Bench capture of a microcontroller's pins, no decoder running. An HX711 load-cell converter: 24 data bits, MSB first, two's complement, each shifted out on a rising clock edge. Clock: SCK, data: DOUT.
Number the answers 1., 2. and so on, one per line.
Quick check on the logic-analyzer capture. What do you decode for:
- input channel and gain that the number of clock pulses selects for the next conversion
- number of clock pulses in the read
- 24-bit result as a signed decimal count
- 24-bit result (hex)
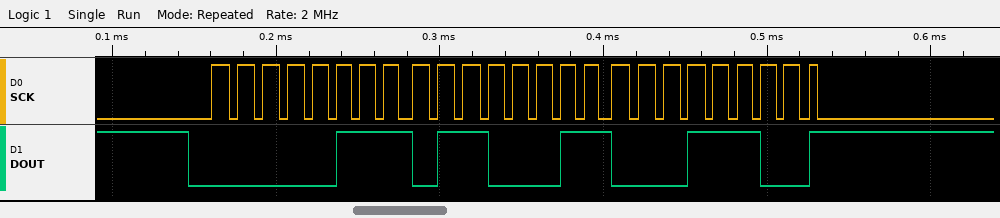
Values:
1. channel A, gain 128
2. 25
3. 484124
4. 0x07631C
